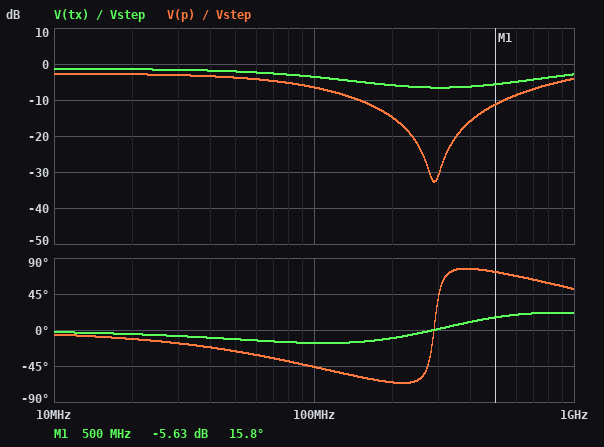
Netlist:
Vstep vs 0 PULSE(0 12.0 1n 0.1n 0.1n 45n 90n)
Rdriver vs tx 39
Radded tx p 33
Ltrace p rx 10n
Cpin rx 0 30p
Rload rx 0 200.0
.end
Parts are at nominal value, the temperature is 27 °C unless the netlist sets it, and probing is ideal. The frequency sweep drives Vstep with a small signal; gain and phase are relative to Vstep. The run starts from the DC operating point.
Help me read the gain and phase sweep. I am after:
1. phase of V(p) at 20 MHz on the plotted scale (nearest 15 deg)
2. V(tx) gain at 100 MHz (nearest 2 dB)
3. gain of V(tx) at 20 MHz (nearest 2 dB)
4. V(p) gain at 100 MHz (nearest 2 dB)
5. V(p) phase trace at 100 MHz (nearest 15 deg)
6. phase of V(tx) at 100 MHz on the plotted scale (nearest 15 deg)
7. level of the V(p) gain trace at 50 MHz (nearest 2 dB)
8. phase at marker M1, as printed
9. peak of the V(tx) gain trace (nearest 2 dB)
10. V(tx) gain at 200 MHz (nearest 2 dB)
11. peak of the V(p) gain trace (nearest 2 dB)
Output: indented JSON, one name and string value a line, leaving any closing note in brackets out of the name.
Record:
{
  "phase of V(p) at 20 MHz on the plotted scale": "-15 deg",
  "V(tx) gain at 100 MHz": "-4 dB",
  "gain of V(tx) at 20 MHz": "-2 dB",
  "V(p) gain at 100 MHz": "-6 dB",
  "V(p) phase trace at 100 MHz": "-45 deg",
  "phase of V(tx) at 100 MHz on the plotted scale": "-15 deg",
  "level of the V(p) gain trace at 50 MHz": "-4 dB",
  "phase at marker M1, as printed": "15.8 deg",
  "peak of the V(tx) gain trace": "-2 dB",
  "V(tx) gain at 200 MHz": "-6 dB",
  "peak of the V(p) gain trace": "-2 dB"
}
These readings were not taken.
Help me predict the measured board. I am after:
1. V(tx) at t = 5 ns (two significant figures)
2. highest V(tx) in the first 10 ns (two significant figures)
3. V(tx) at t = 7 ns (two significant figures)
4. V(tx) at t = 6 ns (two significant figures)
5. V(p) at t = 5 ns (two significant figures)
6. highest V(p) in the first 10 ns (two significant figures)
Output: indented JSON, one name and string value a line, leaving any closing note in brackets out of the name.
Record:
{
  "V(tx) at t = 5 ns": "9.9 V",
  "highest V(tx) in the first 10 ns": "10 V",
  "V(tx) at t = 7 ns": "10 V",
  "V(tx) at t = 6 ns": "10 V",
  "V(p) at t = 5 ns": "8.1 V",
  "highest V(p) in the first 10 ns": "8.8 V"
}
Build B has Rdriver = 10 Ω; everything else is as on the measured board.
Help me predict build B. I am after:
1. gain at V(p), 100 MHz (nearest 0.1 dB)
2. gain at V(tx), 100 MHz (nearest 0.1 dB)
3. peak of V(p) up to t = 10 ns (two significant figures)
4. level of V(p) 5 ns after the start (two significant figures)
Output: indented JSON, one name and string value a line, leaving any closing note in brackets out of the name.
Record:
{
  "gain at V(p), 100 MHz": "-3.9 dB",
  "gain at V(tx), 100 MHz": "-1.0 dB",
  "peak of V(p) up to t = 10 ns": "9.9 V",
  "level of V(p) 5 ns after the start": "9.7 V"
}
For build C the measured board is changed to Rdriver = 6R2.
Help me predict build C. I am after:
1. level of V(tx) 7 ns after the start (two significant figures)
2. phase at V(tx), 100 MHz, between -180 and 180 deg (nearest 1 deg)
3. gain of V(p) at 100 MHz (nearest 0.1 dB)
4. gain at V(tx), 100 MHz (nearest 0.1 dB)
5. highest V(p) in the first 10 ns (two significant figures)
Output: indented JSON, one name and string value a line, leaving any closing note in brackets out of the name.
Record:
{
  "level of V(tx) 7 ns after the start": "12 V",
  "phase at V(tx), 100 MHz, between -180 and 180 deg": "-4 deg",
  "gain of V(p) at 100 MHz": "-3.5 dB",
  "gain at V(tx), 100 MHz": "-0.6 dB",
  "highest V(p) in the first 10 ns": "10 V"
}
